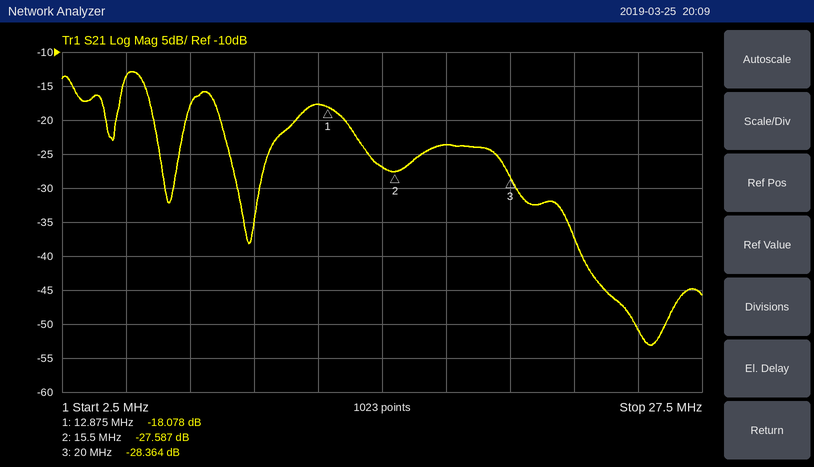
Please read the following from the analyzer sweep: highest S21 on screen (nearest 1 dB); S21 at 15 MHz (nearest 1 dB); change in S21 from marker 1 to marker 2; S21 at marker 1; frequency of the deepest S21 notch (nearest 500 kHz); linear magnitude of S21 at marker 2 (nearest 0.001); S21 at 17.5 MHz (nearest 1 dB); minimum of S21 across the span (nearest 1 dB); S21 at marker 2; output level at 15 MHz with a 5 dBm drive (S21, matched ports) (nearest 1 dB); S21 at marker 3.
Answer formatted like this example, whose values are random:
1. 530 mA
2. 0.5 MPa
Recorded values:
1. -13 dB
2. -27 dB
3. -9.509 dB
4. -18.078 dB
5. 25.5 MHz
6. 0.042
7. -24 dB
8. -53 dB
9. -27.587 dB
10. -22 dBm
11. -28.364 dB
